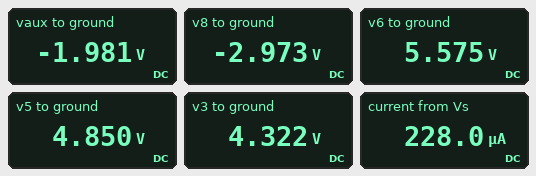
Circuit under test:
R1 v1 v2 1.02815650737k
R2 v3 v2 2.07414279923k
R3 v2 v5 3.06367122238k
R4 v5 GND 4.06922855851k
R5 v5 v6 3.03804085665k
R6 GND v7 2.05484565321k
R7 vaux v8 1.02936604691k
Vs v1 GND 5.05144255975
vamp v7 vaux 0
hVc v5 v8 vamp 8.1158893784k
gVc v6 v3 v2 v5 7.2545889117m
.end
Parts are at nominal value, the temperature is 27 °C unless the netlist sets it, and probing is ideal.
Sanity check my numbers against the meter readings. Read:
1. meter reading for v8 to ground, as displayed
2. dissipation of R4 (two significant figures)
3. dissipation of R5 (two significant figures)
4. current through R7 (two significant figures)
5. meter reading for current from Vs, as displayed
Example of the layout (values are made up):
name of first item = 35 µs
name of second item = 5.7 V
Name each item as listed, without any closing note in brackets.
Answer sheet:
meter reading for v8 to ground, as displayed = -2.973 V
dissipation of R4 = 5.8 mW
dissipation of R5 = 170 µW
current through R7 = 960 µA
meter reading for current from Vs, as displayed = 228.0 µA
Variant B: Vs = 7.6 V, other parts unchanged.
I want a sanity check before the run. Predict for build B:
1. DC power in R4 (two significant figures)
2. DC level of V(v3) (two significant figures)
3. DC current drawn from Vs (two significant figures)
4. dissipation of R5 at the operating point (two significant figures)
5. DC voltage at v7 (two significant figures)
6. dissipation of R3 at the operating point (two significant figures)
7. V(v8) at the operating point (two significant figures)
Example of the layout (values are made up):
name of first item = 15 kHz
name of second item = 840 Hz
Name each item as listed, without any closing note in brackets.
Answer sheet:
DC power in R4 = 13 mW
DC level of V(v3) = 6.5 V
DC current drawn from Vs = 340 µA
dissipation of R5 at the operating point = 390 µW
DC voltage at v7 = -3.0 V
dissipation of R3 at the operating point = 800 nW
V(v8) at the operating point = -4.5 V
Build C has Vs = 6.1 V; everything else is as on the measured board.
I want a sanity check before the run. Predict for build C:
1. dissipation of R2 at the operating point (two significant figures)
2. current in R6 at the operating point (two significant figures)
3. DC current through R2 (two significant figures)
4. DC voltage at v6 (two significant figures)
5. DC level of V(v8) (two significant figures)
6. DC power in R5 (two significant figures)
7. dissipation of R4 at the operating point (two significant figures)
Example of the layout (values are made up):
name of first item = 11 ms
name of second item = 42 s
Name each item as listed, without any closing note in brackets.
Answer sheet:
dissipation of R2 at the operating point = 170 µW
current in R6 at the operating point = 1.2 mA
DC current through R2 = 290 µA
DC voltage at v6 = 6.7 V
DC level of V(v8) = -3.6 V
DC power in R5 = 250 µW
dissipation of R4 at the operating point = 8.4 mW
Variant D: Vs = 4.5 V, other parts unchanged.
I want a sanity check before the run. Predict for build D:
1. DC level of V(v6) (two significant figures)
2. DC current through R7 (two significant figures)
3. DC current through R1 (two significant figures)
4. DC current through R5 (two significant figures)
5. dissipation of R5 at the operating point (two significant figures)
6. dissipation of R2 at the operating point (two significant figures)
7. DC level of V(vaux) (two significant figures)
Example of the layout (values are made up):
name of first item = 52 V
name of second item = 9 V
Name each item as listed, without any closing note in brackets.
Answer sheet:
DC level of V(v6) = 5.0 V
DC current through R7 = 860 µA
DC current through R1 = 200 µA
DC current through R5 = 210 µA
dissipation of R5 at the operating point = 140 µW
dissipation of R2 at the operating point = 94 µW
DC level of V(vaux) = -1.8 V
